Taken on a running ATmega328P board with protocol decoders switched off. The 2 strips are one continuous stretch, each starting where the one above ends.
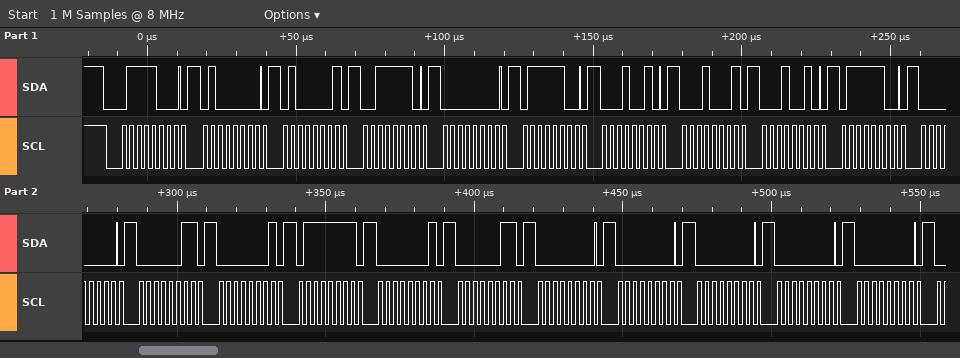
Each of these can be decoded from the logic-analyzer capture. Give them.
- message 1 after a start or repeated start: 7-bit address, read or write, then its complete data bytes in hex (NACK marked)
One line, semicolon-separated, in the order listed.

0x3C write: 40 41 3E 00 7C 12 11 12 7C 00 03 01 7F 01 03 00 00 00 00 00
